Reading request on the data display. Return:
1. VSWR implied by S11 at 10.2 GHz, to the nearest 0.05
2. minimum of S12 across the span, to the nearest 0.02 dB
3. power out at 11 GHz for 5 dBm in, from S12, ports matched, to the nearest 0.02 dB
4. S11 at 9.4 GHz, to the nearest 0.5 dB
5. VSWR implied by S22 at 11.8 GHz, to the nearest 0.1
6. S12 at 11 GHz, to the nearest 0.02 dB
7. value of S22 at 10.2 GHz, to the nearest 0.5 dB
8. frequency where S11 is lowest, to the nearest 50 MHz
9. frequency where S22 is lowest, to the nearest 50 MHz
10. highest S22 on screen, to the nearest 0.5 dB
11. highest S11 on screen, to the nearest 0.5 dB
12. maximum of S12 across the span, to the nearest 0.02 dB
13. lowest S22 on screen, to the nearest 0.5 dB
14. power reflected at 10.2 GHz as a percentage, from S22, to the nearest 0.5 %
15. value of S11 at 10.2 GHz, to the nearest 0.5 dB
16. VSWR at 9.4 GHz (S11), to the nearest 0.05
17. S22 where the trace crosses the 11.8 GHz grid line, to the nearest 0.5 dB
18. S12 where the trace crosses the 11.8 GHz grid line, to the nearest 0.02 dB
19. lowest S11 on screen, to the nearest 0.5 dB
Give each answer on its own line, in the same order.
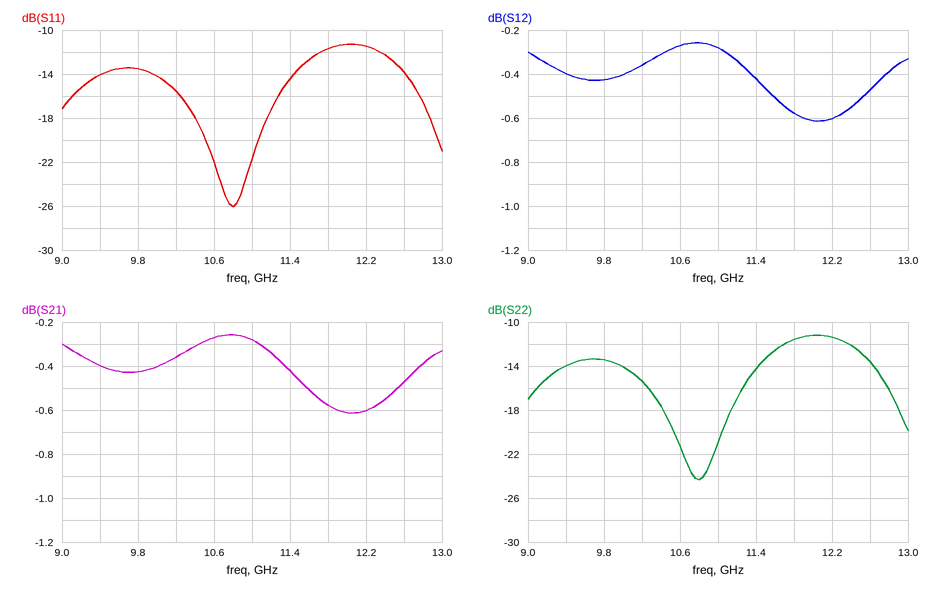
1.40
-0.62 dB
4.72 dBm
-14.0 dB
1.7
-0.28 dB
-15.5 dB
10.80 GHz
10.80 GHz
-11.0 dB
-11.5 dB
-0.26 dB
-24.5 dB
3.0 %
-15.5 dB
1.50
-11.5 dB
-0.58 dB
-26.0 dB
